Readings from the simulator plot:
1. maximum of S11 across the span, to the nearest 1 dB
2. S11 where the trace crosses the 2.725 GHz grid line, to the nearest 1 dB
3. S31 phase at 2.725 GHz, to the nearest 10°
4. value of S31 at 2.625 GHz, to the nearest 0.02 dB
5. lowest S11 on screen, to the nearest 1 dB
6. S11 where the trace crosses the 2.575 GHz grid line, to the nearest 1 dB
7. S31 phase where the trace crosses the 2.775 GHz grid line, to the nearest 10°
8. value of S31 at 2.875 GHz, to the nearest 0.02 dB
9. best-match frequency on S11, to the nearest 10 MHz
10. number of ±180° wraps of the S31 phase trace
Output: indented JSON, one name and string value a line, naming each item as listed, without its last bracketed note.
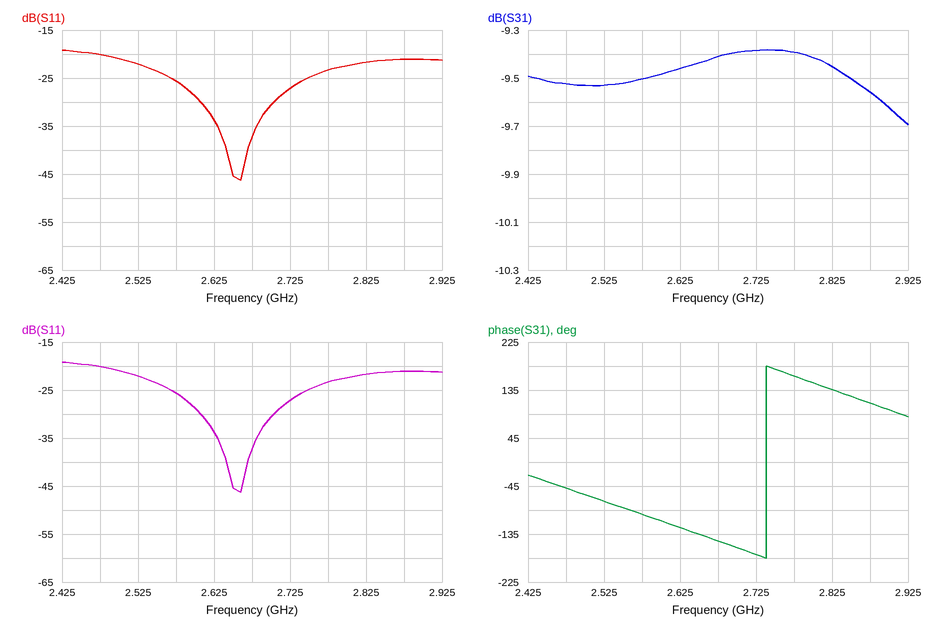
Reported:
{
  "maximum of S11 across the span, to the nearest 1 dB": "-19 dB",
  "S11 where the trace crosses the 2.725 GHz grid line, to the nearest 1 dB": "-27 dB",
  "S31 phase at 2.725 GHz, to the nearest 10°": "-170°",
  "value of S31 at 2.625 GHz, to the nearest 0.02 dB": "-9.46 dB",
  "lowest S11 on screen, to the nearest 1 dB": "-46 dB",
  "S11 where the trace crosses the 2.575 GHz grid line, to the nearest 1 dB": "-26 dB",
  "S31 phase where the trace crosses the 2.775 GHz grid line, to the nearest 10°": "160°",
  "value of S31 at 2.875 GHz, to the nearest 0.02 dB": "-9.56 dB",
  "best-match frequency on S11, to the nearest 10 MHz": "2.66 GHz",
  "number of ±180° wraps of the S31 phase trace": "1"
}
